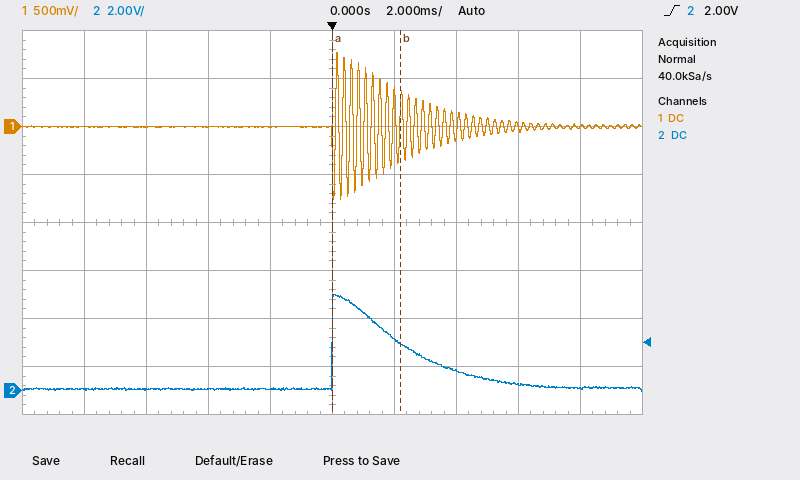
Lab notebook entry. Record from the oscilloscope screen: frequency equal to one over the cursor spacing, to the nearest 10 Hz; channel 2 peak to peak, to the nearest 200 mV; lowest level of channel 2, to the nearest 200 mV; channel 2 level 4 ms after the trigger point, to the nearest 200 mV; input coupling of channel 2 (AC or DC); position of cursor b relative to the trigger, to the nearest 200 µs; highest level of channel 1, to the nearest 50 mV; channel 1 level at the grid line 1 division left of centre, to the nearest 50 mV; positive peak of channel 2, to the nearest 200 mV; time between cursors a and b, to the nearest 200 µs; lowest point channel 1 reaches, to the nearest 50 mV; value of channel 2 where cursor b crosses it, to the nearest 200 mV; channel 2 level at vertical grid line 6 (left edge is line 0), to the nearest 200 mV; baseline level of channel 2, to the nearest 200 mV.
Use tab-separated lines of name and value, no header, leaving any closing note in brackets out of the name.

frequency equal to one over the cursor spacing, to the nearest 10 Hz	450 Hz
channel 2 peak to peak, to the nearest 200 mV	4.0 V
lowest level of channel 2, to the nearest 200 mV	0.0 V
channel 2 level 4 ms after the trigger point, to the nearest 200 mV	800 mV
input coupling of channel 2	DC
position of cursor b relative to the trigger, to the nearest 200 µs	+2.2 ms
highest level of channel 1, to the nearest 50 mV	750 mV
channel 1 level at the grid line 1 division left of centre, to the nearest 50 mV	0 mV
positive peak of channel 2, to the nearest 200 mV	4.0 V
time between cursors a and b, to the nearest 200 µs	2.2 ms
lowest point channel 1 reaches, to the nearest 50 mV	-750 mV
value of channel 2 where cursor b crosses it, to the nearest 200 mV	2.0 V
channel 2 level at vertical grid line 6 (left edge is line 0), to the nearest 200 mV	2.2 V
baseline level of channel 2, to the nearest 200 mV	0.0 V
